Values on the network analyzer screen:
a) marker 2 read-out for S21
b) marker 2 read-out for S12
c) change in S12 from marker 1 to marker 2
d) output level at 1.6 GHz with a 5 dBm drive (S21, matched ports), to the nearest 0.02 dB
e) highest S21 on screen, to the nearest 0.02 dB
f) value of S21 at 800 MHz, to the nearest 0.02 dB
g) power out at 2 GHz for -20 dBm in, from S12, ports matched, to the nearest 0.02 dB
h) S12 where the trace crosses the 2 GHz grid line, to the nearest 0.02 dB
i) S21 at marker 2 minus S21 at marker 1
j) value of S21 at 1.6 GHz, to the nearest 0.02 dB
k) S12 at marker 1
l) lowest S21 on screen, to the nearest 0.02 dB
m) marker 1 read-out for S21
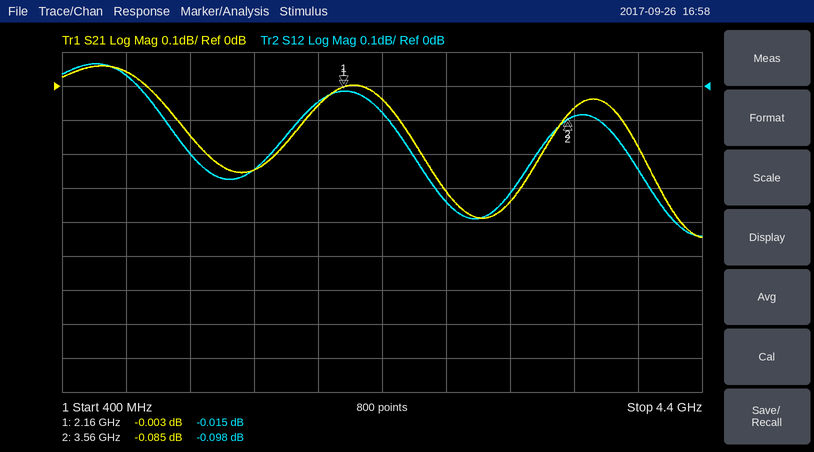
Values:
-0.085 dB
-0.098 dB
-0.083 dB
4.76 dBm
0.06 dB
0.04 dB
-20.04 dBm
-0.04 dB
-0.082 dB
-0.24 dB
-0.015 dB
-0.44 dB
-0.003 dB
